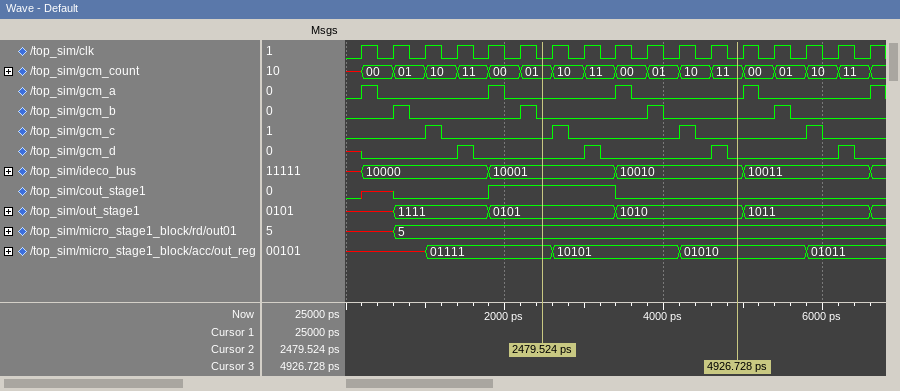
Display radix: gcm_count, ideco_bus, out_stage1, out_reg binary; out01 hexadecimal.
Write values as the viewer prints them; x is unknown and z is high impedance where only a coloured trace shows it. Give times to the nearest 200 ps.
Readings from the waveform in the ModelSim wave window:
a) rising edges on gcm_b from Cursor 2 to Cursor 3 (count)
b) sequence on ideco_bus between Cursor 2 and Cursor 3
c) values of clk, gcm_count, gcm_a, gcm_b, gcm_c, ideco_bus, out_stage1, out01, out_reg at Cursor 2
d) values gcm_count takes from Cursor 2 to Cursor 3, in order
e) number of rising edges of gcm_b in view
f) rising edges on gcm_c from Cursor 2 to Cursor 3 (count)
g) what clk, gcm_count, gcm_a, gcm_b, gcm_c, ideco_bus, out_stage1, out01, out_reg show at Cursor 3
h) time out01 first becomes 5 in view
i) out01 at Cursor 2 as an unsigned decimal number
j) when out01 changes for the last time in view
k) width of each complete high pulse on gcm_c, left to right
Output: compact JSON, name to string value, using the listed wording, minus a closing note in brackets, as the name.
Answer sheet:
{"rising edges on gcm_b from Cursor 2 to Cursor 3": "1", "sequence on ideco_bus between Cursor 2 and Cursor 3": "10001, 10010", "values of clk, gcm_count, gcm_a, gcm_b, gcm_c, ideco_bus, out_stage1, out01, out_reg at Cursor 2": "clk=0, gcm_count=01, gcm_a=0, gcm_b=0, gcm_c=0, ideco_bus=10001, out_stage1=0101, out01=5, out_reg=01111", "values gcm_count takes from Cursor 2 to Cursor 3, in order": "01, 10, 11, 00, 01, 10, 11", "number of rising edges of gcm_b in view": "4", "rising edges on gcm_c from Cursor 2 to Cursor 3": "2", "what clk, gcm_count, gcm_a, gcm_b, gcm_c, ideco_bus, out_stage1, out01, out_reg show at Cursor 3": "clk=0, gcm_count=11, gcm_a=0, gcm_b=0, gcm_c=0, ideco_bus=10010, out_stage1=1010, out01=5, out_reg=01010", "time out01 first becomes 5 in view": "600 ps", "out01 at Cursor 2 as an unsigned decimal number": "5", "when out01 changes for the last time in view": "600 ps", "width of each complete high pulse on gcm_c, left to right": "200 ps, 200 ps, 200 ps, 200 ps"}
